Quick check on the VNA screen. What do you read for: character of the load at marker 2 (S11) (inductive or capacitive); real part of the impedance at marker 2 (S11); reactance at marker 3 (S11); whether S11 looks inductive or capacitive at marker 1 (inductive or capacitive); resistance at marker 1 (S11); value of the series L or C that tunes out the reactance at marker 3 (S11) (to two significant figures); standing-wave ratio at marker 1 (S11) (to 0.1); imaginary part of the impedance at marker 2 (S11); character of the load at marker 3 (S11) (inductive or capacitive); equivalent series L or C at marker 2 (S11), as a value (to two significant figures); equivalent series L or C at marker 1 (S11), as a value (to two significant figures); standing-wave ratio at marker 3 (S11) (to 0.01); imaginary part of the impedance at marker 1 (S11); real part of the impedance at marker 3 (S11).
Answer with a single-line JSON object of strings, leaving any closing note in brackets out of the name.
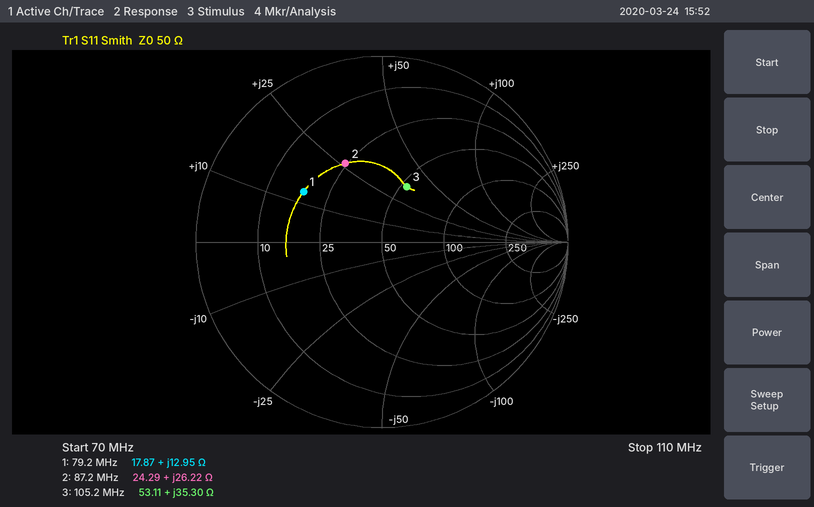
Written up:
{"character of the load at marker 2 (S11)": "inductive", "real part of the impedance at marker 2": "24.29 Ω", "reactance at marker 3": "+35.30 Ω", "whether S11 looks inductive or capacitive at marker 1": "inductive", "resistance at marker 1": "17.87 Ω", "value of the series L or C that tunes out the reactance at marker 3 (S11)": "43 pF", "standing-wave ratio at marker 1 (S11)": "3.0", "imaginary part of the impedance at marker 2": "+26.22 Ω", "character of the load at marker 3 (S11)": "inductive", "equivalent series L or C at marker 2 (S11), as a value": "48 nH", "equivalent series L or C at marker 1 (S11), as a value": "26 nH", "standing-wave ratio at marker 3 (S11)": "1.96", "imaginary part of the impedance at marker 1": "+12.95 Ω", "real part of the impedance at marker 3": "53.11 Ω"}
